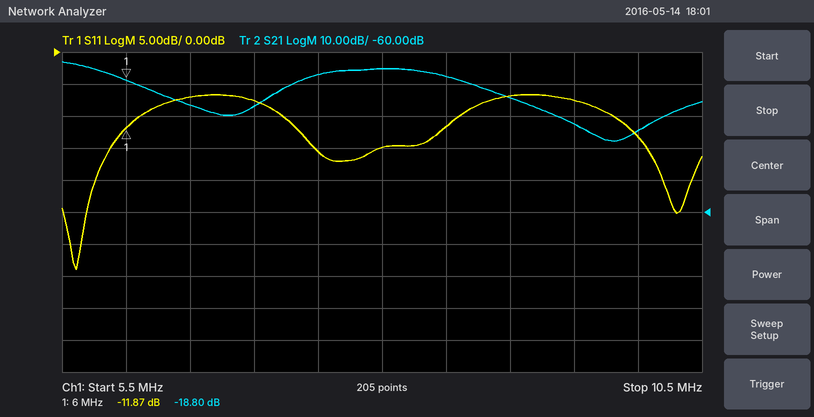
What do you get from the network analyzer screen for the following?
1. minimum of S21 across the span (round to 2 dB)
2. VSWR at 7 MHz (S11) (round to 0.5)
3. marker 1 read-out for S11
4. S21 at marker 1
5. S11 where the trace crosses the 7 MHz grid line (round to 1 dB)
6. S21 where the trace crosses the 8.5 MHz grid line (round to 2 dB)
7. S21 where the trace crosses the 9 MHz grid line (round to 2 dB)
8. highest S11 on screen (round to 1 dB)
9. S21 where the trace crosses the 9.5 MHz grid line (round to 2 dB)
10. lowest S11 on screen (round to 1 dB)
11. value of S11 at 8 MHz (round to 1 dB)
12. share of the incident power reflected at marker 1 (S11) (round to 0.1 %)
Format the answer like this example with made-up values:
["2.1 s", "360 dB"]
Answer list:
["-38 dB", "2.5", "-11.87 dB", "-18.80 dB", "-8 dB", "-18 dB", "-24 dB", "-7 dB", "-32 dB", "-34 dB", "-15 dB", "6.5 %"]
